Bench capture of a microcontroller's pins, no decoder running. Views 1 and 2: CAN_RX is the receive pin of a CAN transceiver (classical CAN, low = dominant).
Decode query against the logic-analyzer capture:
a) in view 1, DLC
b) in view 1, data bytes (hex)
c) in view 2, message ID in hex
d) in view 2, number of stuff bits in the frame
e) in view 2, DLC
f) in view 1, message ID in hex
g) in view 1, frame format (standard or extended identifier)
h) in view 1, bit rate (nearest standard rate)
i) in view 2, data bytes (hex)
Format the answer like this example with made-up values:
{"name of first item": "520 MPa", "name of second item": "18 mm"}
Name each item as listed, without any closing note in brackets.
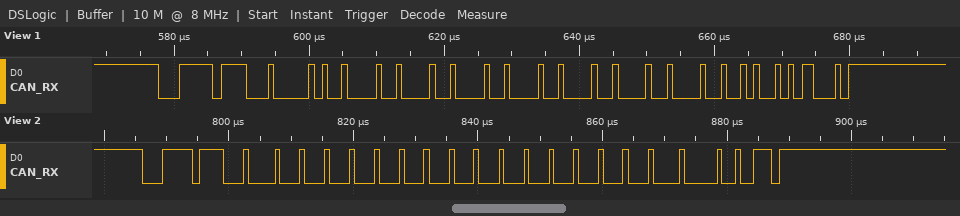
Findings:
{"in view 1, DLC": "8", "in view 1, data bytes": "12 12 12 12 12 12 12 12", "in view 2, message ID in hex": "0x1FF", "in view 2, number of stuff bits in the frame": "2", "in view 2, DLC": "8", "in view 1, message ID in hex": "0x1FF", "in view 1, frame format": "standard", "in view 1, bit rate": "1000 kbit/s", "in view 2, data bytes": "44 44 44 44 44 44 44 44"}
